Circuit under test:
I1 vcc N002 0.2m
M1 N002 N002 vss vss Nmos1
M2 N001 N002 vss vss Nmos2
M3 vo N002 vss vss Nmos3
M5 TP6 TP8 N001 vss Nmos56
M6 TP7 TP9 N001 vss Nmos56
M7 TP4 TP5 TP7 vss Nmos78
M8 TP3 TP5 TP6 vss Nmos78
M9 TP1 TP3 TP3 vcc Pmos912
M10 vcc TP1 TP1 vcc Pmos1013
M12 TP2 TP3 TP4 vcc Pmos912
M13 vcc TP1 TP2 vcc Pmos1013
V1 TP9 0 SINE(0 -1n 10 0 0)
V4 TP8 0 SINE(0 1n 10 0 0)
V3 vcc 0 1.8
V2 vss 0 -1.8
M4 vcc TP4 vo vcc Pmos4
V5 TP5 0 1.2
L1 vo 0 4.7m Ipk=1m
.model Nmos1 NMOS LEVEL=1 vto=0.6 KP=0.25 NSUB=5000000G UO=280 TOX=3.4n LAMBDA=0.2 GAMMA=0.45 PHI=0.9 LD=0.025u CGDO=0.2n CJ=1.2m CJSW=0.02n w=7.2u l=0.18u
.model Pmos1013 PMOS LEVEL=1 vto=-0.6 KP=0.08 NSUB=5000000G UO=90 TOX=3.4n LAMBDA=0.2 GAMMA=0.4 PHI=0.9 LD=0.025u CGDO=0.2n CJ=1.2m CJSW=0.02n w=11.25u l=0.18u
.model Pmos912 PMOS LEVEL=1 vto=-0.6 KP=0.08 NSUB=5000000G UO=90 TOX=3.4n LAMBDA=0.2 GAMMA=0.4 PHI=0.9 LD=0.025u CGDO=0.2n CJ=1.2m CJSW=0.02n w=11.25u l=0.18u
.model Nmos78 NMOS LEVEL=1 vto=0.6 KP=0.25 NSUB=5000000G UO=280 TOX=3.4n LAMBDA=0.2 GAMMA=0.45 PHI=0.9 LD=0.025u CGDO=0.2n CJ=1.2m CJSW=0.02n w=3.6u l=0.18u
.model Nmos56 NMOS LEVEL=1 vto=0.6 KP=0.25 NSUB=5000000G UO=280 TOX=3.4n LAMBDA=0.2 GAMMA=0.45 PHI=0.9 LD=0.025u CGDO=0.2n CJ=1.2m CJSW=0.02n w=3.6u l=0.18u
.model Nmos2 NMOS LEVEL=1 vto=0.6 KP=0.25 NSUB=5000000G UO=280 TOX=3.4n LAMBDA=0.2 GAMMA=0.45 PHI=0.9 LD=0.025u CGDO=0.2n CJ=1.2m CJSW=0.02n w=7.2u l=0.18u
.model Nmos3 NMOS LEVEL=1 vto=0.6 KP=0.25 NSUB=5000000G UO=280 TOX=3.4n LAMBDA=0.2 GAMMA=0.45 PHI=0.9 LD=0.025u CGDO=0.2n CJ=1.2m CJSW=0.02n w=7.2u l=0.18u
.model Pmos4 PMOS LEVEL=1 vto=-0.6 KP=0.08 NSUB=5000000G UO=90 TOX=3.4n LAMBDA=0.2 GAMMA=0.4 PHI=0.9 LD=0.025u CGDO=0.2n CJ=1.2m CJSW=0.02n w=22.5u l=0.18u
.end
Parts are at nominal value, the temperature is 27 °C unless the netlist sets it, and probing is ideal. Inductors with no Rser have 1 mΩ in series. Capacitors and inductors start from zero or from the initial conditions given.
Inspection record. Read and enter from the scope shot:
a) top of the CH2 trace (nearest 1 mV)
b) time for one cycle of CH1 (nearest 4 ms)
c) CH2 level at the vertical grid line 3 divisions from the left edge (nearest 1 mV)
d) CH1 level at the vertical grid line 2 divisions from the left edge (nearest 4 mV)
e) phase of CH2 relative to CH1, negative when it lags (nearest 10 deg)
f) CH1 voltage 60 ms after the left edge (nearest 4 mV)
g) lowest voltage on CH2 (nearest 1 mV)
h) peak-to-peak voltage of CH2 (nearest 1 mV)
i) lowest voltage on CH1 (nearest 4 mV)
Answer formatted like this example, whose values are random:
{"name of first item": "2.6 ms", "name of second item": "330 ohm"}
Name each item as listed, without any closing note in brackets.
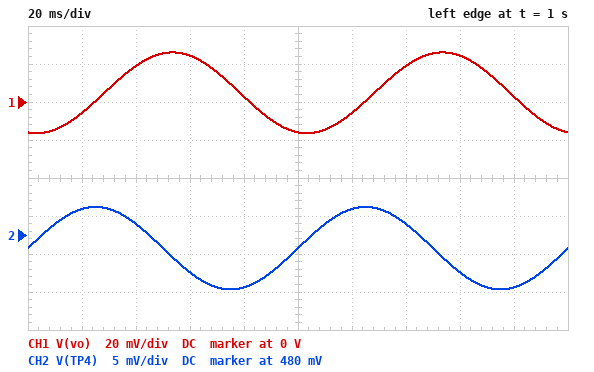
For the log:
{"top of the CH2 trace": "484 mV", "time for one cycle of CH1": "100 ms", "CH2 level at the vertical grid line 3 divisions from the left edge": "475 mV", "CH1 level at the vertical grid line 2 divisions from the left edge": "20 mV", "phase of CH2 relative to CH1, negative when it lags": "100 deg", "CH1 voltage 60 ms after the left edge": "24 mV", "lowest voltage on CH2": "473 mV", "peak-to-peak voltage of CH2": "11 mV", "lowest voltage on CH1": "-16 mV"}
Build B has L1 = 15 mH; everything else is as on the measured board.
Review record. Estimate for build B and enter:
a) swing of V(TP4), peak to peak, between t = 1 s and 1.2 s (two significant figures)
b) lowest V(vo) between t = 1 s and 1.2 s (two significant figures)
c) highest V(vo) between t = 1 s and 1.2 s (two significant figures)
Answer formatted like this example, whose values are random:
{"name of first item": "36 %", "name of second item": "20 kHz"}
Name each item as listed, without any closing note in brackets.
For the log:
{"swing of V(TP4), peak to peak, between t = 1 s and 1.2 s": "11 mV", "lowest V(vo) between t = 1 s and 1.2 s": "-53 mV", "highest V(vo) between t = 1 s and 1.2 s": "62 mV"}
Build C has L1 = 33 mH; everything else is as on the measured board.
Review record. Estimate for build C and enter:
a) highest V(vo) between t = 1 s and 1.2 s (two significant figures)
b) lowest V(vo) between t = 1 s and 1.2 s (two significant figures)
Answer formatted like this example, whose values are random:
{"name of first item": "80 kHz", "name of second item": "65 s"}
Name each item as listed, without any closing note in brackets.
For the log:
{"highest V(vo) between t = 1 s and 1.2 s": "89 mV", "lowest V(vo) between t = 1 s and 1.2 s": "-80 mV"}
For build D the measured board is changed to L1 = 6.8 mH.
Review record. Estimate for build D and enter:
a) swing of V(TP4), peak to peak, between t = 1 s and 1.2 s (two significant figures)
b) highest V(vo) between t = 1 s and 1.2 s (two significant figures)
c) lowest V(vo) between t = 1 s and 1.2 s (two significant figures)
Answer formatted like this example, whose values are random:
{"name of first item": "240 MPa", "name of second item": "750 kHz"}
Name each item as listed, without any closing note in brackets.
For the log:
{"swing of V(TP4), peak to peak, between t = 1 s and 1.2 s": "11 mV", "highest V(vo) between t = 1 s and 1.2 s": "35 mV", "lowest V(vo) between t = 1 s and 1.2 s": "-25 mV"}
